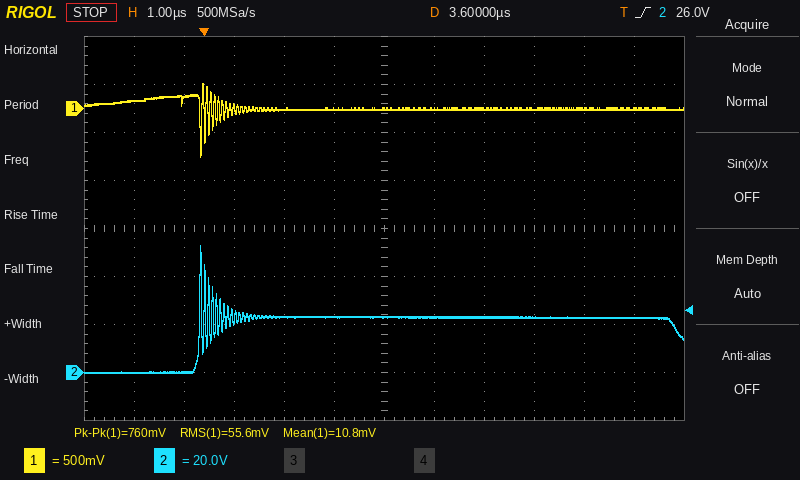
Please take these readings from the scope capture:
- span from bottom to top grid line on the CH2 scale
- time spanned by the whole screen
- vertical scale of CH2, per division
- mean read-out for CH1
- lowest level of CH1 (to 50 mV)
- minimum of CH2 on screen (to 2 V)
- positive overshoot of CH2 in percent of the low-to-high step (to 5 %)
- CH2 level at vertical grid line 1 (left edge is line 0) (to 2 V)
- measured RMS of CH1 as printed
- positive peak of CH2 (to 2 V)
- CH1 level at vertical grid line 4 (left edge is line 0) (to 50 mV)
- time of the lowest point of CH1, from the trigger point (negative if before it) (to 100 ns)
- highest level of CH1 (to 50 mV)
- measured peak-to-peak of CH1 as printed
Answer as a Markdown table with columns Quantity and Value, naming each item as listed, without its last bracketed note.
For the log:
| Quantity | Value |
|---|---|
| span from bottom to top grid line on the CH2 scale | 160 V |
| time spanned by the whole screen | 12 µs |
| vertical scale of CH2, per division | 20 V |
| mean read-out for CH1 | 10.8 mV |
| lowest level of CH1 | -500 mV |
| minimum of CH2 on screen | 0 V |
| positive overshoot of CH2 in percent of the low-to-high step | 130 % |
| CH2 level at vertical grid line 1 (left edge is line 0) | 0 V |
| measured RMS of CH1 as printed | 55.6 mV |
| positive peak of CH2 | 52 V |
| CH1 level at vertical grid line 4 (left edge is line 0) | 0 mV |
| time of the lowest point of CH1, from the trigger point (negative if before it) | -100 ns |
| highest level of CH1 | 250 mV |
| measured peak-to-peak of CH1 as printed | 760 mV |
